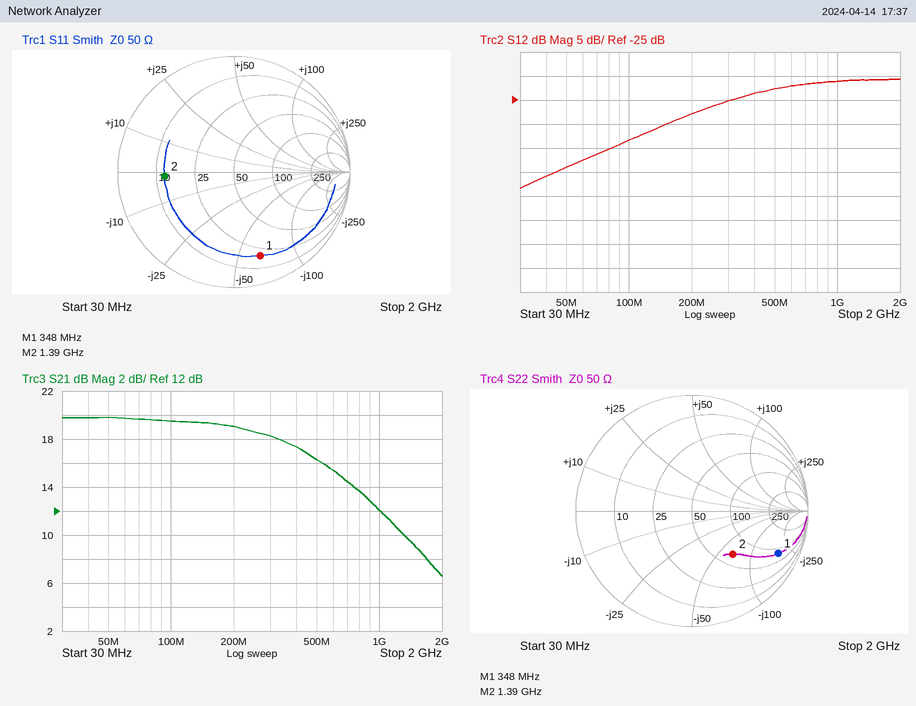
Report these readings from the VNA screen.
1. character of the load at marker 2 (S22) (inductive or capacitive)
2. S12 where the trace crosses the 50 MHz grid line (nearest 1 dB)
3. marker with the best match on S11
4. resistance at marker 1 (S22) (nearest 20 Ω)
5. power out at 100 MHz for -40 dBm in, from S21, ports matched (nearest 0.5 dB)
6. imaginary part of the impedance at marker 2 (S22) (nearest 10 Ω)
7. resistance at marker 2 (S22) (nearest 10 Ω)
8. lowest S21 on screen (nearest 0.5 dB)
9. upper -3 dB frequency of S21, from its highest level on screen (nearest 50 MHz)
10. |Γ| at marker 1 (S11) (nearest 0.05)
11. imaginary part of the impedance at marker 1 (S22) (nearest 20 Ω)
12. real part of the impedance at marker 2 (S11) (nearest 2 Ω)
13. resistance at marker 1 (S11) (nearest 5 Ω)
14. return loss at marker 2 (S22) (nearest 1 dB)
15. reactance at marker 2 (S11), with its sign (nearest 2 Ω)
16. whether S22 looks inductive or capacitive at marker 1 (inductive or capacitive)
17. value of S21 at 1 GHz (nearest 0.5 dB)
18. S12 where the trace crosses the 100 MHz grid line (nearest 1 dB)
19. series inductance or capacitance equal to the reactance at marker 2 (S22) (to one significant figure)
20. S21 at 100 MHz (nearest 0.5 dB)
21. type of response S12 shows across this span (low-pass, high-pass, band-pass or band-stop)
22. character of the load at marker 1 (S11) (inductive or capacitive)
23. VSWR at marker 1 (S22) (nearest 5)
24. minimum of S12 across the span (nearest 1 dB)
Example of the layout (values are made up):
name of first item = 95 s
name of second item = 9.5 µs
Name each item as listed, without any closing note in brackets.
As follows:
character of the load at marker 2 (S22) = capacitive
S12 where the trace crosses the 50 MHz grid line = -39 dB
marker with the best match on S11 = marker 2
resistance at marker 1 (S22) = 80 Ω
power out at 100 MHz for -40 dBm in, from S21, ports matched = -20.5 dBm
imaginary part of the impedance at marker 2 (S22) = -70 Ω
resistance at marker 2 (S22) = 70 Ω
lowest S21 on screen = 6.5 dB
upper -3 dB frequency of S21, from its highest level on screen = 450 MHz
|Γ| at marker 1 (S11) = 0.75
imaginary part of the impedance at marker 1 (S22) = -180 Ω
real part of the impedance at marker 2 (S11) = 12 Ω
resistance at marker 1 (S11) = 20 Ω
return loss at marker 2 (S22) = 6 dB
reactance at marker 2 (S11), with its sign = -2 Ω
whether S22 looks inductive or capacitive at marker 1 = capacitive
value of S21 at 1 GHz = 12.0 dB
S12 where the trace crosses the 100 MHz grid line = -33 dB
series inductance or capacitance equal to the reactance at marker 2 (S22) = 2 pF
S21 at 100 MHz = 19.5 dB
type of response S12 shows across this span = high-pass
character of the load at marker 1 (S11) = capacitive
VSWR at marker 1 (S22) = 10
minimum of S12 across the span = -43 dB
